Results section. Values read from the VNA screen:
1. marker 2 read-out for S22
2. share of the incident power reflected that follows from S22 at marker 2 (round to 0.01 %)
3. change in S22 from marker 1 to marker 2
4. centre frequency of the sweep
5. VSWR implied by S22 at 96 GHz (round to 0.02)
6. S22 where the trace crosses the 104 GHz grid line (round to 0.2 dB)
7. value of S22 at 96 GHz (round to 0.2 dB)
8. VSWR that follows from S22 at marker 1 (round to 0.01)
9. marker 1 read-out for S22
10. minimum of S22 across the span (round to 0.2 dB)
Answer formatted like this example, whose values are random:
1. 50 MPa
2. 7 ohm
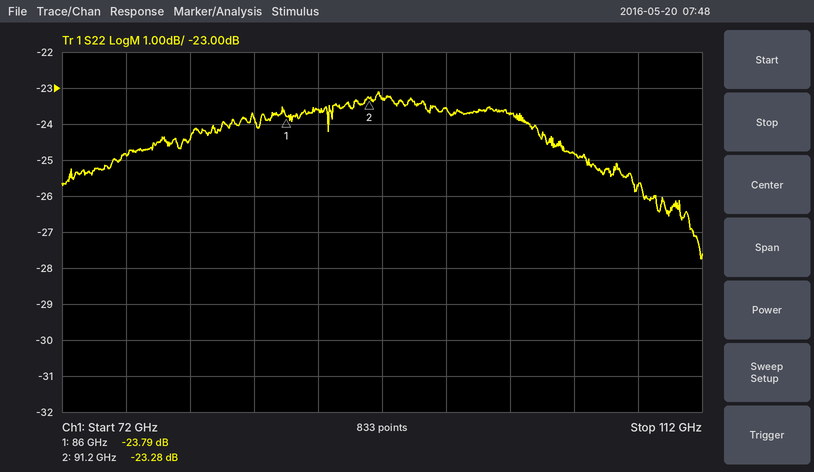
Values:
1. -23.28 dB
2. 0.47 %
3. 0.51 dB
4. 92 GHz
5. 1.14
6. -24.8 dB
7. -23.6 dB
8. 1.14
9. -23.79 dB
10. -27.8 dB
